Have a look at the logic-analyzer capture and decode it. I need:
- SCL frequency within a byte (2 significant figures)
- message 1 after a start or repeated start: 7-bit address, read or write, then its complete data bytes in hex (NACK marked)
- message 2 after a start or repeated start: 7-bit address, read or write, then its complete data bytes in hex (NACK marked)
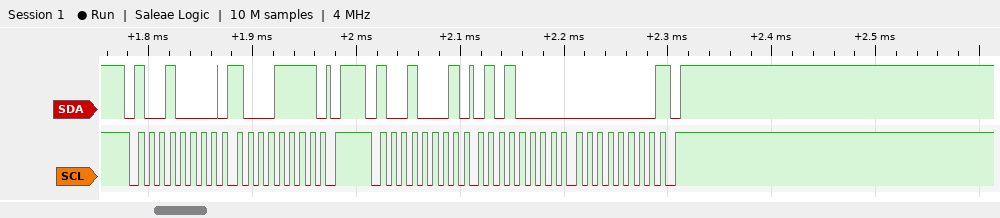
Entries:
100 kHz
0x48 write: 8F
0x48 read: 50 00 NACK
